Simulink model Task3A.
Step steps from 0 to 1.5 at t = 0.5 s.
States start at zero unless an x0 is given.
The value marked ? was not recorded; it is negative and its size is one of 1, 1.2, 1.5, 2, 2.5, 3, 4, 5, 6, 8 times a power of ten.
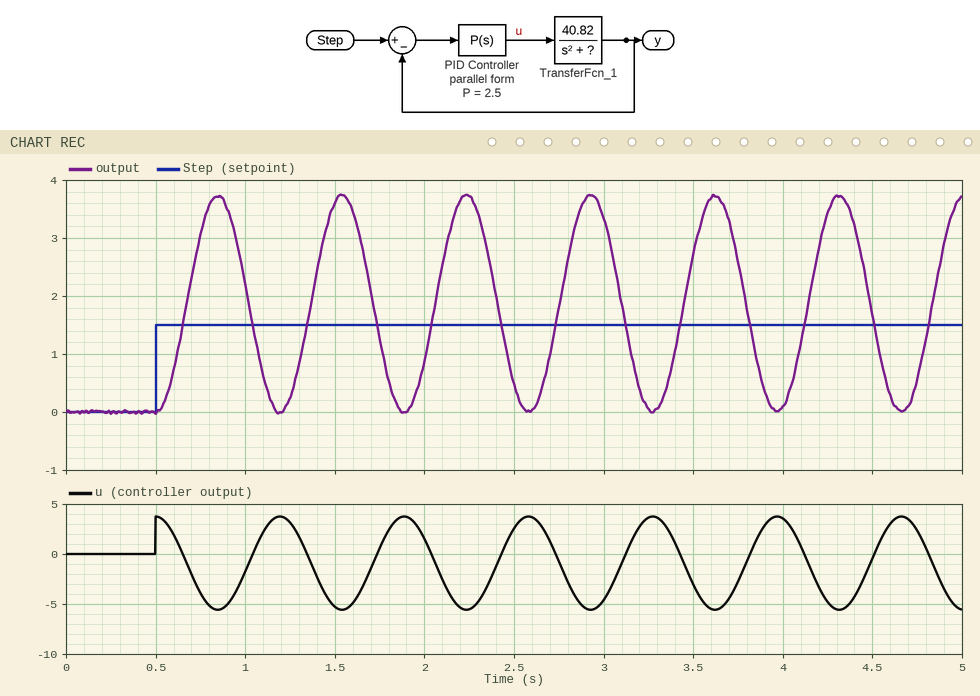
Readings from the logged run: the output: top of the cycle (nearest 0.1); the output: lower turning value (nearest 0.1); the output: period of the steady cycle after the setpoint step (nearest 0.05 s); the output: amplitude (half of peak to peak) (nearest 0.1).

3.7
0.0
0.70 s
1.9
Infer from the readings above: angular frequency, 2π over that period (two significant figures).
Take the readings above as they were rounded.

9.0 rad/s
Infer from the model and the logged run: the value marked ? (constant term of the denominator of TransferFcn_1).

-20
